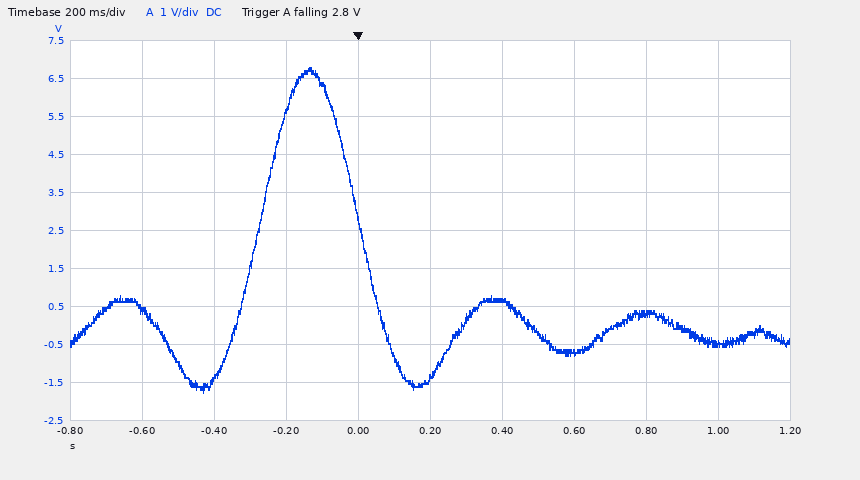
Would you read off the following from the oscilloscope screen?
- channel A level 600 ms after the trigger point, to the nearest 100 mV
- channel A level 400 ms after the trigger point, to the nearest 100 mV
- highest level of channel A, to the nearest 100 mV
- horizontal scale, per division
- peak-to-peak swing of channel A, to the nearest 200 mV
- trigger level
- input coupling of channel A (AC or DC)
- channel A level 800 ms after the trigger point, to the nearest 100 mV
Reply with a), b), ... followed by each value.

a) -700 mV
b) 700 mV
c) 6.8 V
d) 200 ms
e) 8.6 V
f) 2.8 V
g) DC
h) 300 mV
